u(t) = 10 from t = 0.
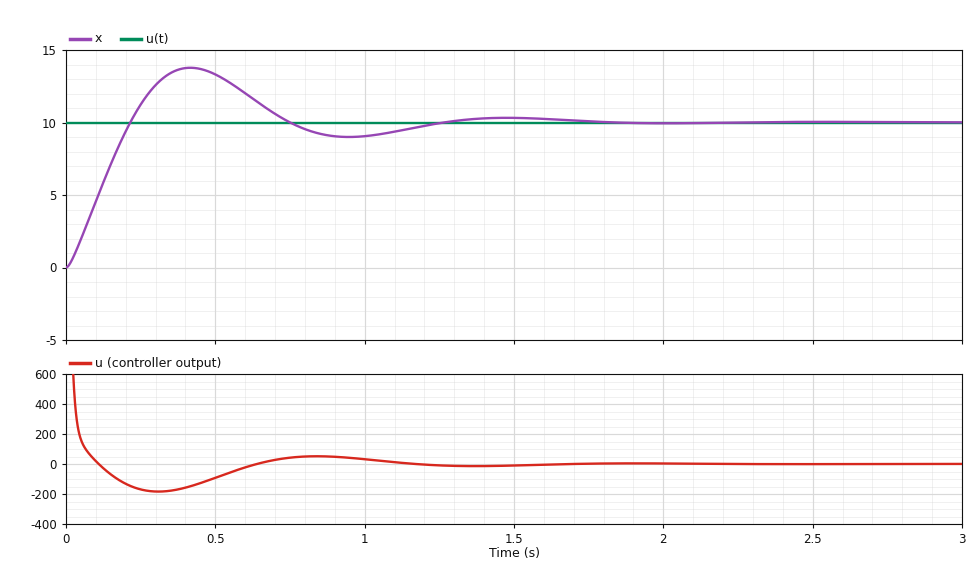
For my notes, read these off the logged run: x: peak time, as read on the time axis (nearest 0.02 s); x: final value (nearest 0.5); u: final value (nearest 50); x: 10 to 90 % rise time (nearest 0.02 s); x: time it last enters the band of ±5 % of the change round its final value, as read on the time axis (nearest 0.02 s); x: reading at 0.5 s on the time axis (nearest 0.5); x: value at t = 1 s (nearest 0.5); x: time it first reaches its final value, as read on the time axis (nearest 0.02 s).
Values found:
0.42 s
10.0
0
0.16 s
1.14 s
13.5
9.0
0.22 s
